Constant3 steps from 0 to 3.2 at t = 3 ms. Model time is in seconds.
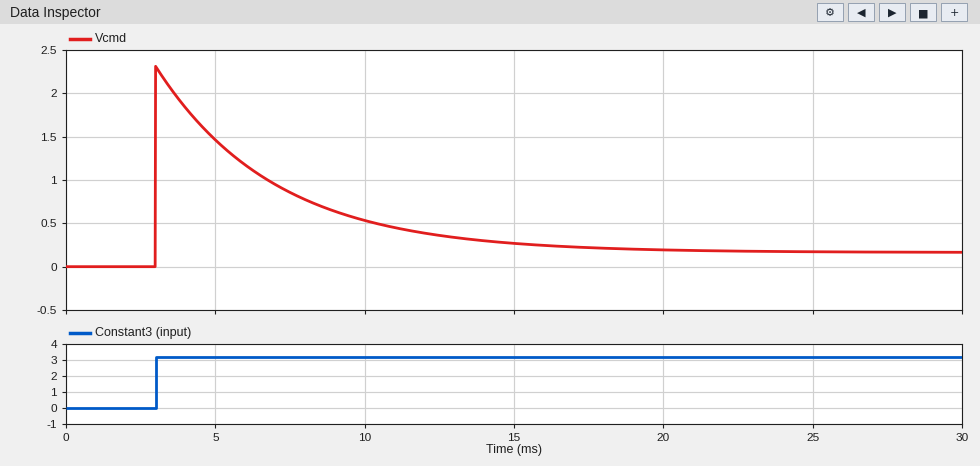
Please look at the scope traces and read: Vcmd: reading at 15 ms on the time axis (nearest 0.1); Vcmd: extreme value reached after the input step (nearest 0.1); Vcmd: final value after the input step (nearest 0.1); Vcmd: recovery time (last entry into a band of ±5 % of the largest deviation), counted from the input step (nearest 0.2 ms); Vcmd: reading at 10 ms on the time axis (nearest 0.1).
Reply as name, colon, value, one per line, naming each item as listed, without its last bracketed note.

Vcmd: reading at 15 ms on the time axis: 0.3
Vcmd: extreme value reached after the input step: 2.3
Vcmd: final value after the input step: 0.2
Vcmd: recovery time (last entry into a band of ±5 % of the largest deviation), counted from the input step: 11.6 ms
Vcmd: reading at 10 ms on the time axis: 0.5
